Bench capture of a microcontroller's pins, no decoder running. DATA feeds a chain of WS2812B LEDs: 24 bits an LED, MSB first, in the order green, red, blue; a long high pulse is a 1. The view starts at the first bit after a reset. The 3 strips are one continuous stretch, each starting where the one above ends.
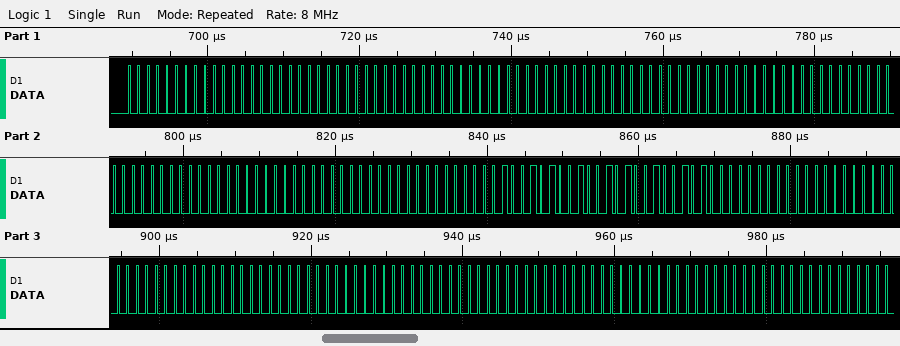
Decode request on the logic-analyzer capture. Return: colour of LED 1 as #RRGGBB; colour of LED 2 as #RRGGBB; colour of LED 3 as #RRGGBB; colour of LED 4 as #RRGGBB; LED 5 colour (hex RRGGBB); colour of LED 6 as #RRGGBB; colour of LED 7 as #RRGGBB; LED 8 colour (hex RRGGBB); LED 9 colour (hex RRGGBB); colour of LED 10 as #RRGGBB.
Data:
#000000
#000000
#000000
#000000
#000000
#252525
#000000
#000000
#000000
#000000
